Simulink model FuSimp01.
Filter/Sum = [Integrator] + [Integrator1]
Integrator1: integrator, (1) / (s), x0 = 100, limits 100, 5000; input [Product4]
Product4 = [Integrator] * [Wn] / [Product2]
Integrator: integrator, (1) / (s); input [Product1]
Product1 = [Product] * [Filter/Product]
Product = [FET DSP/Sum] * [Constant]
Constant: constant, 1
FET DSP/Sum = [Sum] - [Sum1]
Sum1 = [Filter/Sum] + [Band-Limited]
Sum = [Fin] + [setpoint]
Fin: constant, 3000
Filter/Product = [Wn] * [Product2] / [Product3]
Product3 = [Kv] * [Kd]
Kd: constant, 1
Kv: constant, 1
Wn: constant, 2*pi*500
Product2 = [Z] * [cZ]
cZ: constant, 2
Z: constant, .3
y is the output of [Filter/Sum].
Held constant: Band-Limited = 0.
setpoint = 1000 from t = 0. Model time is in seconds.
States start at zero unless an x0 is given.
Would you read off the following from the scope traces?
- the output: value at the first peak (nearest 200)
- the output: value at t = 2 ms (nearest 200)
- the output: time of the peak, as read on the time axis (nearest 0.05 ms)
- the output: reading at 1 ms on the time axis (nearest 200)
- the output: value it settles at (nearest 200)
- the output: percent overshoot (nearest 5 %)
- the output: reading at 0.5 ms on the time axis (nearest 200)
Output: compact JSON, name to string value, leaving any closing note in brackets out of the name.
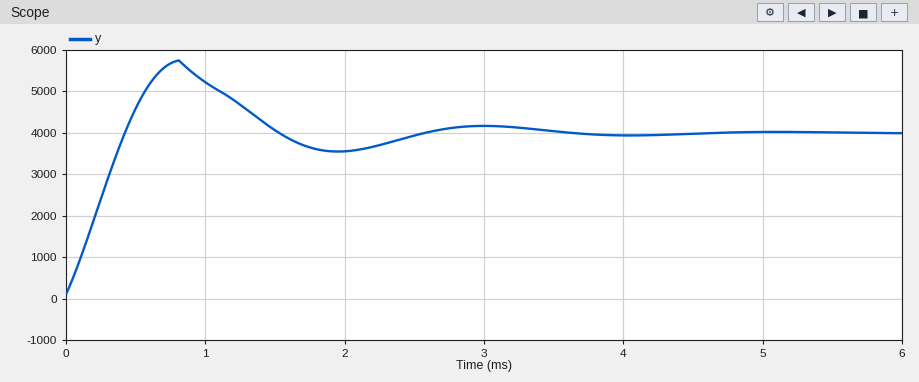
{"the output: value at the first peak": "5800", "the output: value at t = 2 ms": "3600", "the output: time of the peak, as read on the time axis": "0.80 ms", "the output: reading at 1 ms on the time axis": "5200", "the output: value it settles at": "4000", "the output: percent overshoot": "45 %", "the output: reading at 0.5 ms on the time axis": "4600"}
